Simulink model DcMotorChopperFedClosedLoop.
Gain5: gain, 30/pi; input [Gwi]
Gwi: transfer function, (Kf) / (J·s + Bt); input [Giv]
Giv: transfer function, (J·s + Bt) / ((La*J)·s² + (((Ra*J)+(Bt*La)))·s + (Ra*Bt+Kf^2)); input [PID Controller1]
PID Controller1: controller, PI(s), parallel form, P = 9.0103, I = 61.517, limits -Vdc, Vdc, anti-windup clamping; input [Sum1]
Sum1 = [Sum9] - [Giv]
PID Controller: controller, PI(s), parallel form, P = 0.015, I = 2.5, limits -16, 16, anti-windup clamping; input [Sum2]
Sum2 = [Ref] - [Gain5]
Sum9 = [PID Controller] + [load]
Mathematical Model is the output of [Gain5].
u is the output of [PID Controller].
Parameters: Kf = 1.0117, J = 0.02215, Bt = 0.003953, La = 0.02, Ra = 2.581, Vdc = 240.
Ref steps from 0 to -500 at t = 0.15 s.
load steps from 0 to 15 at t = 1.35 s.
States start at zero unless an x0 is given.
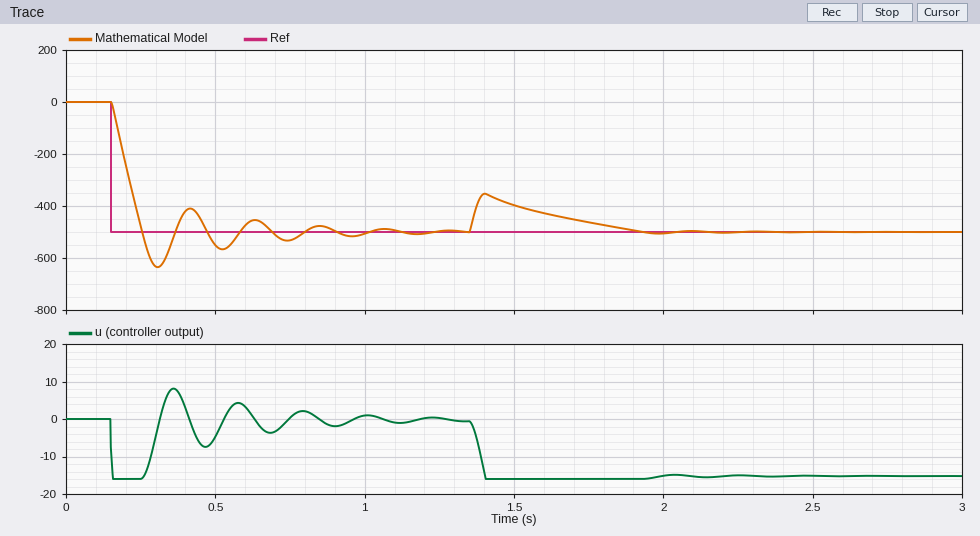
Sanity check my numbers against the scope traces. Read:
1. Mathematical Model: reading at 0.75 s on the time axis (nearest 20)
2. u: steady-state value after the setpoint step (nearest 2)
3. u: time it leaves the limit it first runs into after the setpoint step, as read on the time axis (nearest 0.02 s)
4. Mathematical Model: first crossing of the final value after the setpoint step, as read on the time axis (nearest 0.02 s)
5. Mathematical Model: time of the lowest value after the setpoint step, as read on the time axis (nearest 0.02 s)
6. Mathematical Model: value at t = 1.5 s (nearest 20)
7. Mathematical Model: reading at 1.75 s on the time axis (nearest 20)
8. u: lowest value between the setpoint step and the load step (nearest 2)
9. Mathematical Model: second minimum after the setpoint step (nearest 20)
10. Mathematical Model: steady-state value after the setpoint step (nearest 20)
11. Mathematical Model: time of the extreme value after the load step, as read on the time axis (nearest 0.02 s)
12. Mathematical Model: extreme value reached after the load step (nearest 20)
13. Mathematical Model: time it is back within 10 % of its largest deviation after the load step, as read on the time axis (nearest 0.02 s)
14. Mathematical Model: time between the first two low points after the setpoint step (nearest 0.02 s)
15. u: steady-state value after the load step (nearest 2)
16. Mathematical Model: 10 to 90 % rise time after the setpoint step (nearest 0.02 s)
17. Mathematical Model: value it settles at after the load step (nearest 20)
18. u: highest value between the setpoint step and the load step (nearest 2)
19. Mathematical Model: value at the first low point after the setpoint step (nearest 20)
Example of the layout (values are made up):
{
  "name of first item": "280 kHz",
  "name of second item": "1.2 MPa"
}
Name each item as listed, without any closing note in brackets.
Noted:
{
  "Mathematical Model: reading at 0.75 s on the time axis": "-540",
  "u: steady-state value after the setpoint step": "0",
  "u: time it leaves the limit it first runs into after the setpoint step, as read on the time axis": "0.26 s",
  "Mathematical Model: first crossing of the final value after the setpoint step, as read on the time axis": "0.26 s",
  "Mathematical Model: time of the lowest value after the setpoint step, as read on the time axis": "0.30 s",
  "Mathematical Model: value at t = 1.5 s": "-400",
  "Mathematical Model: reading at 1.75 s on the time axis": "-460",
  "u: lowest value between the setpoint step and the load step": "-16",
  "Mathematical Model: second minimum after the setpoint step": "-560",
  "Mathematical Model: steady-state value after the setpoint step": "-500",
  "Mathematical Model: time of the extreme value after the load step, as read on the time axis": "1.40 s",
  "Mathematical Model: extreme value reached after the load step": "-360",
  "Mathematical Model: time it is back within 10 % of its largest deviation after the load step, as read on the time axis": "1.86 s",
  "Mathematical Model: time between the first two low points after the setpoint step": "0.22 s",
  "u: steady-state value after the load step": "-16",
  "Mathematical Model: 10 to 90 % rise time after the setpoint step": "0.08 s",
  "Mathematical Model: value it settles at after the load step": "-500",
  "u: highest value between the setpoint step and the load step": "8",
  "Mathematical Model: value at the first low point after the setpoint step": "-640"
}
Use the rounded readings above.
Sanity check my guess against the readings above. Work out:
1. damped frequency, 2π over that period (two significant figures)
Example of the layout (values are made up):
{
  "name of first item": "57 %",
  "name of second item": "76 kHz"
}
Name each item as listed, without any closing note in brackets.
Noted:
{
  "damped frequency, 2π over that period": "29 rad/s"
}
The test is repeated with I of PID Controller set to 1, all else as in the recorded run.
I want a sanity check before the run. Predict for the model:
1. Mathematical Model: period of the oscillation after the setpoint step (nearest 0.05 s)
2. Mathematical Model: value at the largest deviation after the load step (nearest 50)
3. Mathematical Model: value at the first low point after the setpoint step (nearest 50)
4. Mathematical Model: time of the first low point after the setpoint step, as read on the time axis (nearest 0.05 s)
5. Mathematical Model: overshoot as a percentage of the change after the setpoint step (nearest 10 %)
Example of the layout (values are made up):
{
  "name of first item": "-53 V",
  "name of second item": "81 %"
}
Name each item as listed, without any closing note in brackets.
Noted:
{
  "Mathematical Model: period of the oscillation after the setpoint step": "0.35 s",
  "Mathematical Model: value at the largest deviation after the load step": "-300",
  "Mathematical Model: value at the first low point after the setpoint step": "-700",
  "Mathematical Model: time of the first low point after the setpoint step, as read on the time axis": "0.35 s",
  "Mathematical Model: overshoot as a percentage of the change after the setpoint step": "40 %"
}
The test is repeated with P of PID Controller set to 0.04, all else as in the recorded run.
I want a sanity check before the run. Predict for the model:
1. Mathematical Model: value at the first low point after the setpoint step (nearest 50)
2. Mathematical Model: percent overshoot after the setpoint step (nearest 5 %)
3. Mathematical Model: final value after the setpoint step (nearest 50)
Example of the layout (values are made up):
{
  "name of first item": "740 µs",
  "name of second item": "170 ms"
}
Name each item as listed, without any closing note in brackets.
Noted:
{
  "Mathematical Model: value at the first low point after the setpoint step": "-600",
  "Mathematical Model: percent overshoot after the setpoint step": "20 %",
  "Mathematical Model: final value after the setpoint step": "-500"
}
